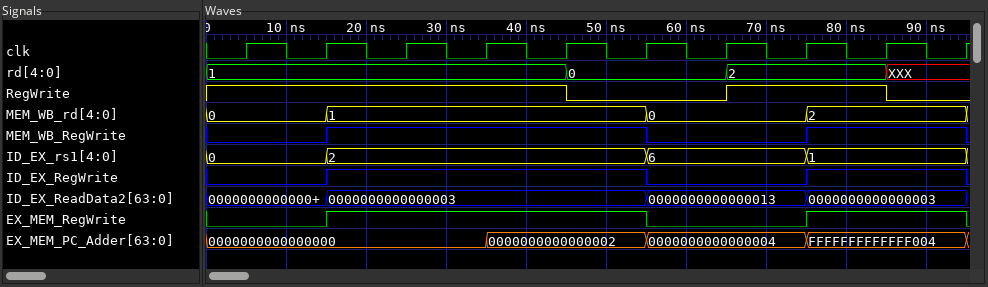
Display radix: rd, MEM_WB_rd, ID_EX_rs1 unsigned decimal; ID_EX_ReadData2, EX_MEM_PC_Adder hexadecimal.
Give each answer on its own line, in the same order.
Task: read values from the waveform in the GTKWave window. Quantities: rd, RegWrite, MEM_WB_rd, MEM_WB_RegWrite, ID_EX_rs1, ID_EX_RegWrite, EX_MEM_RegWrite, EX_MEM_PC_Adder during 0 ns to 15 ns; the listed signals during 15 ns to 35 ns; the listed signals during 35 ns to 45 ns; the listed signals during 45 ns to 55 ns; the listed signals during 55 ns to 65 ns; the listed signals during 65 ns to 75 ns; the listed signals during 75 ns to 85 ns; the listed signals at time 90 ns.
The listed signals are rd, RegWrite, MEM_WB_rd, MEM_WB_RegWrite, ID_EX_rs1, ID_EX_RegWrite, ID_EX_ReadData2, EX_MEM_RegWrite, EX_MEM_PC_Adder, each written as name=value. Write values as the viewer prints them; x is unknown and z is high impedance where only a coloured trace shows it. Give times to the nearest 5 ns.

rd=1, RegWrite=1, MEM_WB_rd=0, MEM_WB_RegWrite=0, ID_EX_rs1=0, ID_EX_RegWrite=0, EX_MEM_RegWrite=0, EX_MEM_PC_Adder=0000000000000000
rd=1, RegWrite=1, MEM_WB_rd=1, MEM_WB_RegWrite=1, ID_EX_rs1=2, ID_EX_RegWrite=1, ID_EX_ReadData2=0000000000000003, EX_MEM_RegWrite=1, EX_MEM_PC_Adder=0000000000000000
rd=1, RegWrite=1, MEM_WB_rd=1, MEM_WB_RegWrite=1, ID_EX_rs1=2, ID_EX_RegWrite=1, ID_EX_ReadData2=0000000000000003, EX_MEM_RegWrite=1, EX_MEM_PC_Adder=0000000000000002
rd=0, RegWrite=0, MEM_WB_rd=1, MEM_WB_RegWrite=1, ID_EX_rs1=2, ID_EX_RegWrite=1, ID_EX_ReadData2=0000000000000003, EX_MEM_RegWrite=1, EX_MEM_PC_Adder=0000000000000002
rd=0, RegWrite=0, MEM_WB_rd=0, MEM_WB_RegWrite=0, ID_EX_rs1=6, ID_EX_RegWrite=0, ID_EX_ReadData2=0000000000000013, EX_MEM_RegWrite=0, EX_MEM_PC_Adder=0000000000000004
rd=2, RegWrite=1, MEM_WB_rd=0, MEM_WB_RegWrite=0, ID_EX_rs1=6, ID_EX_RegWrite=0, ID_EX_ReadData2=0000000000000013, EX_MEM_RegWrite=0, EX_MEM_PC_Adder=0000000000000004
rd=2, RegWrite=1, MEM_WB_rd=2, MEM_WB_RegWrite=1, ID_EX_rs1=1, ID_EX_RegWrite=1, ID_EX_ReadData2=0000000000000003, EX_MEM_RegWrite=1, EX_MEM_PC_Adder=FFFFFFFFFFFFF004
rd=XXX, RegWrite=0, MEM_WB_rd=2, MEM_WB_RegWrite=1, ID_EX_rs1=1, ID_EX_RegWrite=1, ID_EX_ReadData2=0000000000000003, EX_MEM_RegWrite=1, EX_MEM_PC_Adder=FFFFFFFFFFFFF004
